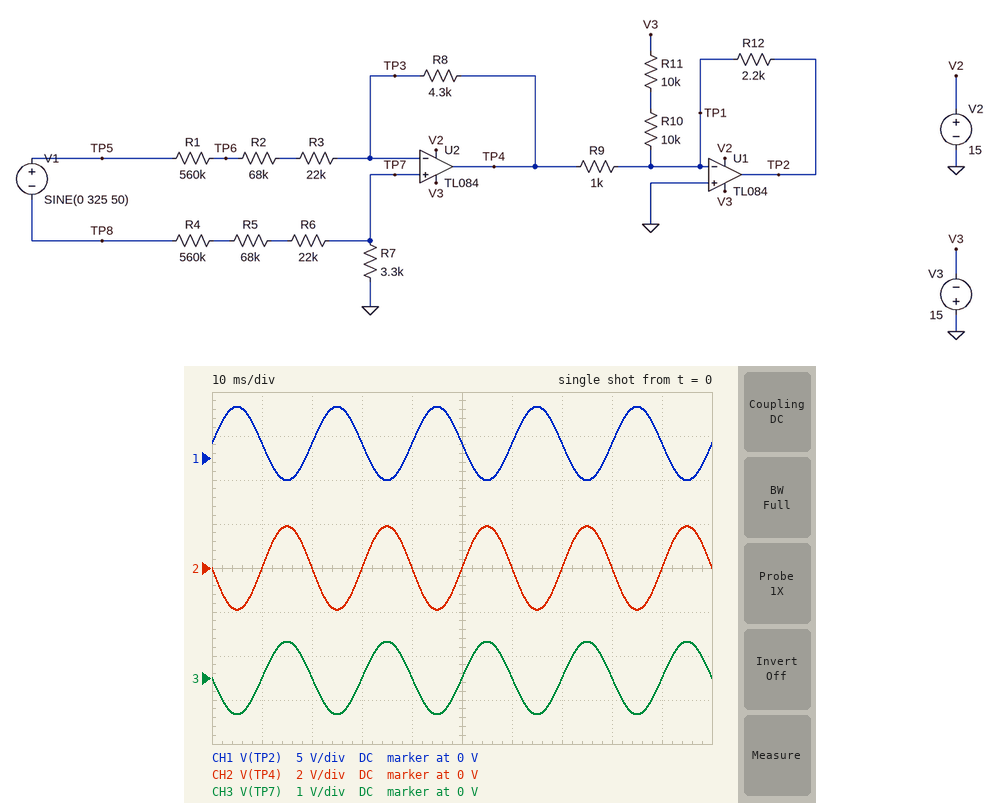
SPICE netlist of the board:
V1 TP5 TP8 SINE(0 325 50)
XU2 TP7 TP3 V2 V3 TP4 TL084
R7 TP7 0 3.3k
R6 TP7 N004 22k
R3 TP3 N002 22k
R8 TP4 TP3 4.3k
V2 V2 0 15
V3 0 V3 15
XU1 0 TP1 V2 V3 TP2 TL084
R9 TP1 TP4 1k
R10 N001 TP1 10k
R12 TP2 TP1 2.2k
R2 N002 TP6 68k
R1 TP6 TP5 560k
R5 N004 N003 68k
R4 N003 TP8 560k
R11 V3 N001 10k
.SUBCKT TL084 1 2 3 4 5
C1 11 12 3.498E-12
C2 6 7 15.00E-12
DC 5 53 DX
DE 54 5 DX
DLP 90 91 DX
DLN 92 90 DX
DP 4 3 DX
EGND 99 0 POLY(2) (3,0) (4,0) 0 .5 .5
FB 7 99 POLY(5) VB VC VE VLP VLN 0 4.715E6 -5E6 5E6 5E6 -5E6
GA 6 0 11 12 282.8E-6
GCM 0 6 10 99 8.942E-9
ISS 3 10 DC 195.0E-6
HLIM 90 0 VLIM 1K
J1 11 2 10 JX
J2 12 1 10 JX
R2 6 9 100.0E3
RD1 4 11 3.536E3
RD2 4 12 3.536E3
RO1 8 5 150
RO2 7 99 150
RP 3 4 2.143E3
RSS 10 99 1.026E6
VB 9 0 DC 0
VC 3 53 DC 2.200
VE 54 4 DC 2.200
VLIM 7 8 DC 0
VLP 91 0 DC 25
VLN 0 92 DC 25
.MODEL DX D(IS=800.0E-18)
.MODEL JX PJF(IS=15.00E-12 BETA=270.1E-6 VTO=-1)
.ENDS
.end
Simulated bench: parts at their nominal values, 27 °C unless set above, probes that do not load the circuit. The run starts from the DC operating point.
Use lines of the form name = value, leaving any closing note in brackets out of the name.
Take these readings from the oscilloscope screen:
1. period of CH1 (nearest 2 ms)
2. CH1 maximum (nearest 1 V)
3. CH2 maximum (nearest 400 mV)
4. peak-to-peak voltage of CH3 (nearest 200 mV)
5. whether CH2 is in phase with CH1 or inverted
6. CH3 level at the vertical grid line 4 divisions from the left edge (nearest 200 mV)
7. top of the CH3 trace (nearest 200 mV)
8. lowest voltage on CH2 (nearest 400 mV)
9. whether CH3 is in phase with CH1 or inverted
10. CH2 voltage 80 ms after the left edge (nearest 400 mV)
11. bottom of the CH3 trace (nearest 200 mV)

period of CH1 = 20 ms
CH1 maximum = 6 V
CH2 maximum = 2.0 V
peak-to-peak voltage of CH3 = 1.6 V
whether CH2 is in phase with CH1 or inverted = inverted
CH3 level at the vertical grid line 4 divisions from the left edge = 0 V
top of the CH3 trace = 800 mV
lowest voltage on CH2 = -2.0 V
whether CH3 is in phase with CH1 or inverted = inverted
CH2 voltage 80 ms after the left edge = 0 V
bottom of the CH3 trace = -800 mV
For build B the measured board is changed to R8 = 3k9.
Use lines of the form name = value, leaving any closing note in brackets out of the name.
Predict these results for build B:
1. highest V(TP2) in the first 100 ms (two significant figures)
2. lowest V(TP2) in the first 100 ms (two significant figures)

highest V(TP2) in the first 100 ms = 5.6 V
lowest V(TP2) in the first 100 ms = -2.3 V
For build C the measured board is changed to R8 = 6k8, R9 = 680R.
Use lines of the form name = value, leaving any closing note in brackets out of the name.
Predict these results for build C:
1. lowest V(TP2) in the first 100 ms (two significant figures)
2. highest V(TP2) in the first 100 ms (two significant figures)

lowest V(TP2) in the first 100 ms = -6.5 V
highest V(TP2) in the first 100 ms = 9.8 V
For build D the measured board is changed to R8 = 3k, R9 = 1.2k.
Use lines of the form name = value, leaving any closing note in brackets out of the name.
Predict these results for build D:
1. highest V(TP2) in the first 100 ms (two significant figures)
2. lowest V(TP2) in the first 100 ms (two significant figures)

highest V(TP2) in the first 100 ms = 4.5 V
lowest V(TP2) in the first 100 ms = -1.2 V
